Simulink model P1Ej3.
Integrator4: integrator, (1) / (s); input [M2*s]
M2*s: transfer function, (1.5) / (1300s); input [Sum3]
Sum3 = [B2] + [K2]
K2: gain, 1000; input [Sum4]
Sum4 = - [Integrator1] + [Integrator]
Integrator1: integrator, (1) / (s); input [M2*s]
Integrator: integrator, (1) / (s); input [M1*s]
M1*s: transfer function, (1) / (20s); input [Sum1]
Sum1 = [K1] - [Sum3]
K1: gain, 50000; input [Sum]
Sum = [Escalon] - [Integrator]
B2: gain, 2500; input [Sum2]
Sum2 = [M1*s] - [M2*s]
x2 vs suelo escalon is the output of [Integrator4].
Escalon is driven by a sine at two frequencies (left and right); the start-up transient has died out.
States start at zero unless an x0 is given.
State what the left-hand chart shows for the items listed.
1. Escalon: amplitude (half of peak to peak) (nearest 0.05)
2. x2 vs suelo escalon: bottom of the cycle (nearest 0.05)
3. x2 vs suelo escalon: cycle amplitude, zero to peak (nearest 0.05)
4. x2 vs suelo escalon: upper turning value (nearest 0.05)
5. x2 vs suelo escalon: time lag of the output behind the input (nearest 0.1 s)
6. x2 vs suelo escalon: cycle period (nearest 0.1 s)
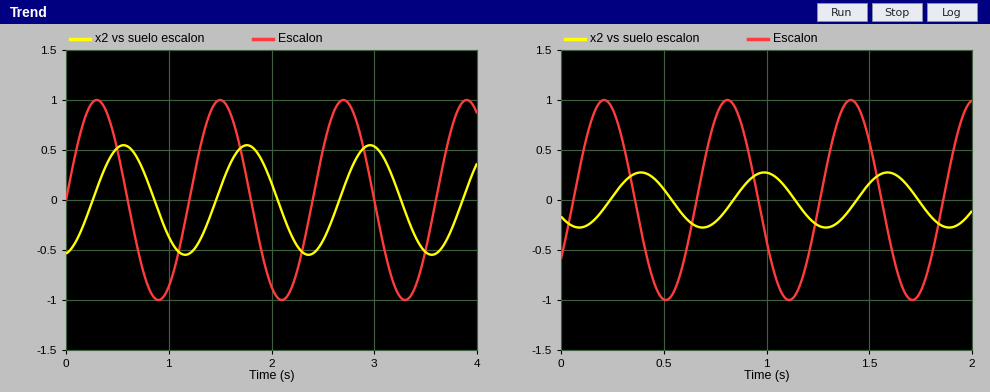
1.00
-0.55
0.55
0.55
0.3 s
1.2 s
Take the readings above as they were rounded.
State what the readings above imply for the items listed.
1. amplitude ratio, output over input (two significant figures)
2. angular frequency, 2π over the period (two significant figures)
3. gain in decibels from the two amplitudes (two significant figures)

0.55
5.2 rad/s
-5.2 dB
